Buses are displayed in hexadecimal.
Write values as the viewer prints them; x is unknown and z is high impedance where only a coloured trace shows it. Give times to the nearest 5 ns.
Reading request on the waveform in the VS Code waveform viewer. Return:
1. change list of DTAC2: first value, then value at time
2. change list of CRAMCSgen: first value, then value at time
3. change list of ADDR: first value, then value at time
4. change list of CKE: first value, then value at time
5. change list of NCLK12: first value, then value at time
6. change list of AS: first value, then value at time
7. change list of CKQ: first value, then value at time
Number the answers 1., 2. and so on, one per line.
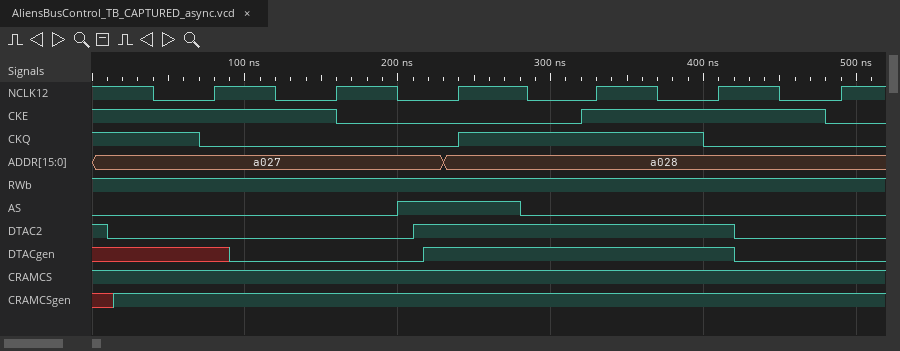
1. 1, 0 at 10 ns, 1 at 210 ns, 0 at 420 ns
2. x, 1 at 15 ns
3. a027, a028 at 230 ns
4. 1, 0 at 160 ns, 1 at 320 ns, 0 at 480 ns
5. 1, 0 at 40 ns, 1 at 80 ns, 0 at 120 ns, 1 at 160 ns, 0 at 200 ns, 1 at 240 ns, 0 at 285 ns, 1 at 330 ns, 0 at 370 ns, 1 at 410 ns, 0 at 450 ns, 1 at 490 ns
6. 0, 1 at 200 ns, 0 at 280 ns
7. 1, 0 at 70 ns, 1 at 240 ns, 0 at 400 ns
